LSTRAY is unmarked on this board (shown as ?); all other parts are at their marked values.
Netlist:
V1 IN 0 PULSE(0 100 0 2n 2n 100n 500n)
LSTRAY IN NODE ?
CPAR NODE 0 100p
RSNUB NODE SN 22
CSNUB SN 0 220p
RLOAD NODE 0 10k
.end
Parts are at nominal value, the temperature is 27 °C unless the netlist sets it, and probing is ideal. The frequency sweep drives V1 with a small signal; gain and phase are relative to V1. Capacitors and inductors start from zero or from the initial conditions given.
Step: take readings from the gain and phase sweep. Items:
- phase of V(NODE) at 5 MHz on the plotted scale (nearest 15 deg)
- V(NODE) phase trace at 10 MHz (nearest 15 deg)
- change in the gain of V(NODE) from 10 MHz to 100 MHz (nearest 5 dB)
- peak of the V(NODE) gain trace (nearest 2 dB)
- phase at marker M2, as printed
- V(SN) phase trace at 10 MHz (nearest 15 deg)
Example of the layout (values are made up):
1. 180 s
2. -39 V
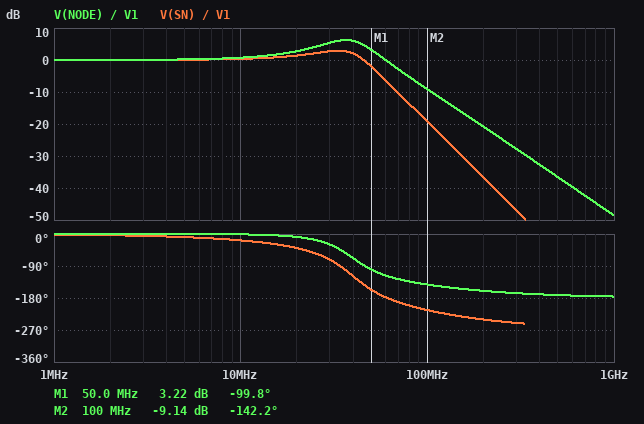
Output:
1. 0 deg
2. 0 deg
3. -10 dB
4. 6 dB
5. -142.2 deg
6. -15 deg
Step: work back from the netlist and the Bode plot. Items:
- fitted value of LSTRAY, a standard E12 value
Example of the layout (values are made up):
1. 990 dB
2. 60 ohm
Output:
1. 68 nH
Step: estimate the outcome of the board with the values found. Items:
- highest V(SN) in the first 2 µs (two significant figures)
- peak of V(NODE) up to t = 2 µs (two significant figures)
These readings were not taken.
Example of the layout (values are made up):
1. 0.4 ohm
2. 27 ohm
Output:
1. 130 V
2. 150 V
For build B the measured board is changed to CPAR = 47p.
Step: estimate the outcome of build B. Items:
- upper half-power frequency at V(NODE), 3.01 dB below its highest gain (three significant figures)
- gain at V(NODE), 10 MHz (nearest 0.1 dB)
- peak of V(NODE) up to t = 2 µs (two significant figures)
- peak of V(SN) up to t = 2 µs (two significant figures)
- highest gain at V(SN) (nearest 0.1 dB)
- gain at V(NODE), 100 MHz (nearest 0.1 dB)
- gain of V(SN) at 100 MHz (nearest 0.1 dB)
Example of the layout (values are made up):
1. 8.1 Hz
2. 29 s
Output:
1. 58.8 MHz
2. 0.6 dB
3. 140 V
4. 120 V
5. 1.1 dB
6. -5.8 dB
7. -15.9 dB
